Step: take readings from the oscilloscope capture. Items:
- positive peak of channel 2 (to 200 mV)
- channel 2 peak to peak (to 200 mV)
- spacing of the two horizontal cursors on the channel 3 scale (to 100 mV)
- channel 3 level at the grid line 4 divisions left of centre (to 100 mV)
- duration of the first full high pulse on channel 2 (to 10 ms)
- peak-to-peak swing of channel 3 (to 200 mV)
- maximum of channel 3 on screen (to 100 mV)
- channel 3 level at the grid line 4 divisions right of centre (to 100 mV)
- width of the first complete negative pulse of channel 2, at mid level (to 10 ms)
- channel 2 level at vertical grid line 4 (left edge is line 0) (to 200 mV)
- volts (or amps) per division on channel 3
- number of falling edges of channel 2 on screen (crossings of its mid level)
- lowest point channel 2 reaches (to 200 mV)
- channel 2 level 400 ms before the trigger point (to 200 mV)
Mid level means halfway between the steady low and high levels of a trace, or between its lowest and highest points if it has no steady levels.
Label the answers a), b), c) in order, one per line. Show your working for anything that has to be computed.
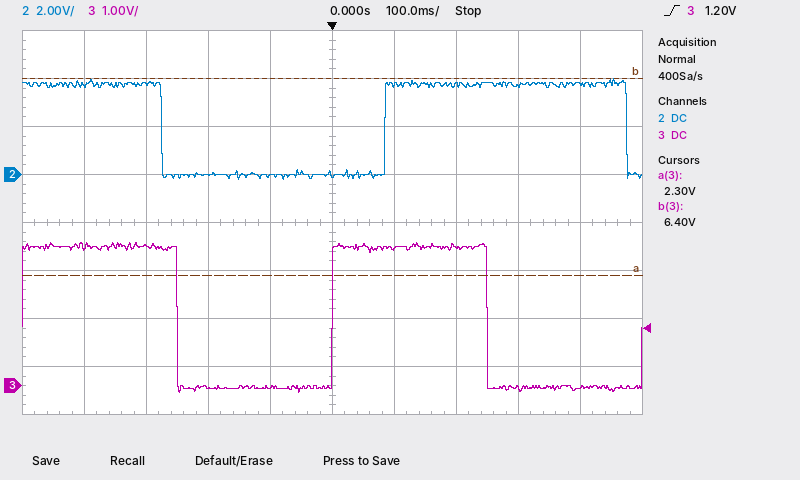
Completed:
a) 4.0 V
b) 4.0 V − (-200 mV) = 4.2 V
c) 4.1 V
d) 2.9 V
e) 390 ms
f) 3.2 V
g) 3.0 V
h) 0.0 V
i) 360 ms
j) 0.0 V
k) 1 V
l) 2
m) -200 mV
n) 3.8 V
